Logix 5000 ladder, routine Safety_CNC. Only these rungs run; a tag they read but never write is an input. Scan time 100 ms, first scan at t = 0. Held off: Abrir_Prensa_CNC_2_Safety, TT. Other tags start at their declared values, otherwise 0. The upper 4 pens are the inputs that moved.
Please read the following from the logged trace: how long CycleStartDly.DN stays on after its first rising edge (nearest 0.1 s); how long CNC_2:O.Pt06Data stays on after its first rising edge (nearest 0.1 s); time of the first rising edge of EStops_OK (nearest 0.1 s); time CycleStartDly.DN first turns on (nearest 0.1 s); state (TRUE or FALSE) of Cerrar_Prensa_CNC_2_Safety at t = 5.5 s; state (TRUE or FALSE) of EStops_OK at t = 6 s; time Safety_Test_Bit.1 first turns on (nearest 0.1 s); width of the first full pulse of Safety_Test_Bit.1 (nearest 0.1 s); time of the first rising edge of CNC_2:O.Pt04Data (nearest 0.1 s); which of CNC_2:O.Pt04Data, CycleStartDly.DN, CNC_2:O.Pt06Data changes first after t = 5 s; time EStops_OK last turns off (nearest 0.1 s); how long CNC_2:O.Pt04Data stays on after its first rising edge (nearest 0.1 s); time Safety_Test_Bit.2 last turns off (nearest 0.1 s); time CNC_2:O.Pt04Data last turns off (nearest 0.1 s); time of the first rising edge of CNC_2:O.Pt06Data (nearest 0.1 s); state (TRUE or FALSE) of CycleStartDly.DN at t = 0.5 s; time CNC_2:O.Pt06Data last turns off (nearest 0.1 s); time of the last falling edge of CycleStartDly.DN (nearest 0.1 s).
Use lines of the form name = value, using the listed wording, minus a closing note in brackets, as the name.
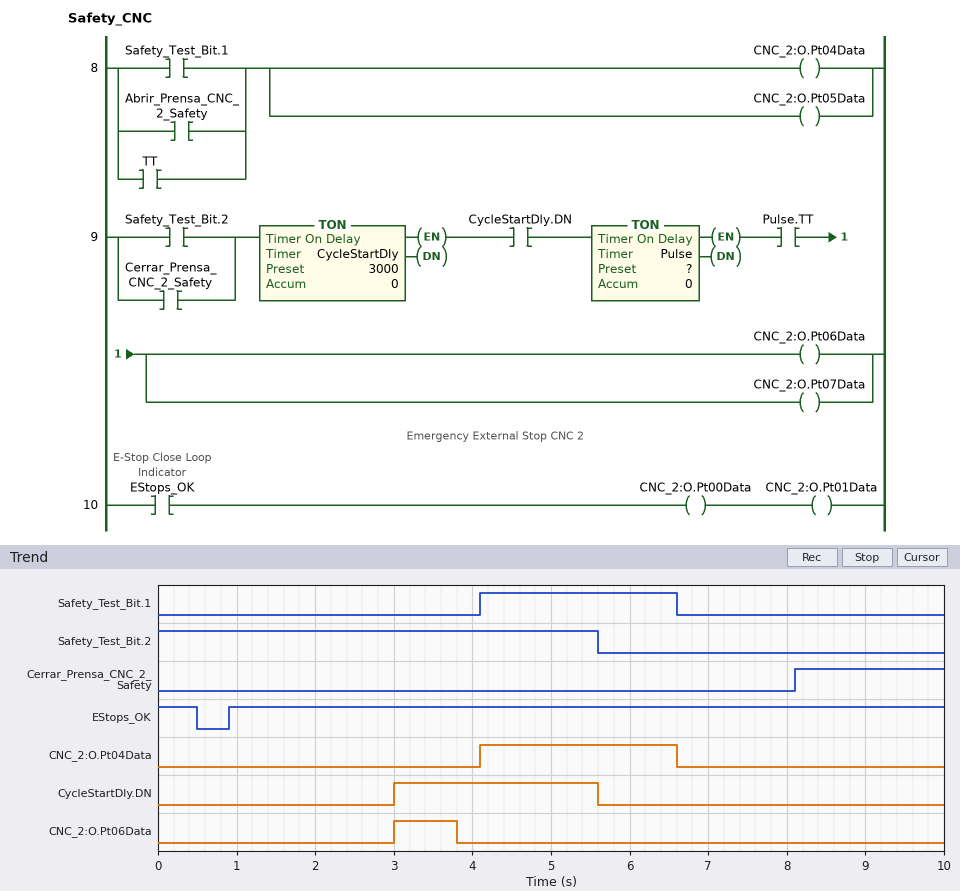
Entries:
how long CycleStartDly.DN stays on after its first rising edge = 2.6 s
how long CNC_2:O.Pt06Data stays on after its first rising edge = 0.8 s
time of the first rising edge of EStops_OK = 0.9 s
time CycleStartDly.DN first turns on = 3.0 s
state (TRUE or FALSE) of Cerrar_Prensa_CNC_2_Safety at t = 5.5 s = FALSE
state (TRUE or FALSE) of EStops_OK at t = 6 s = TRUE
time Safety_Test_Bit.1 first turns on = 4.1 s
width of the first full pulse of Safety_Test_Bit.1 = 2.5 s
time of the first rising edge of CNC_2:O.Pt04Data = 4.1 s
which of CNC_2:O.Pt04Data, CycleStartDly.DN, CNC_2:O.Pt06Data changes first after t = 5 s = CycleStartDly.DN
time EStops_OK last turns off = 0.5 s
how long CNC_2:O.Pt04Data stays on after its first rising edge = 2.5 s
time Safety_Test_Bit.2 last turns off = 5.6 s
time CNC_2:O.Pt04Data last turns off = 6.6 s
time of the first rising edge of CNC_2:O.Pt06Data = 3.0 s
state (TRUE or FALSE) of CycleStartDly.DN at t = 0.5 s = FALSE
time CNC_2:O.Pt06Data last turns off = 3.8 s
time of the last falling edge of CycleStartDly.DN = 5.6 s
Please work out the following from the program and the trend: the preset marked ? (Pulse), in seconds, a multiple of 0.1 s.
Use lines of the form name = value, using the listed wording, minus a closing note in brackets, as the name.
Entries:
the preset marked ? (Pulse), in seconds, a multiple of 0.1 s = 0.8 s
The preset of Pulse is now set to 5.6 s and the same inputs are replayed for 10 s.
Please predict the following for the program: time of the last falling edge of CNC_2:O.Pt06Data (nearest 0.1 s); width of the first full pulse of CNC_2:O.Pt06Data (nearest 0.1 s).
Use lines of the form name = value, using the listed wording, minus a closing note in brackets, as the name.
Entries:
time of the last falling edge of CNC_2:O.Pt06Data = 5.6 s
width of the first full pulse of CNC_2:O.Pt06Data = 2.6 s
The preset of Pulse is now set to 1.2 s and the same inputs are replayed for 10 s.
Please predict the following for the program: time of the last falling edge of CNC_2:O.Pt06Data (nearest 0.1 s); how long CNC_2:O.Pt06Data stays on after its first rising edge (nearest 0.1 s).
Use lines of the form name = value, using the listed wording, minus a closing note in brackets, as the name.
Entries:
time of the last falling edge of CNC_2:O.Pt06Data = 4.2 s
how long CNC_2:O.Pt06Data stays on after its first rising edge = 1.2 s
